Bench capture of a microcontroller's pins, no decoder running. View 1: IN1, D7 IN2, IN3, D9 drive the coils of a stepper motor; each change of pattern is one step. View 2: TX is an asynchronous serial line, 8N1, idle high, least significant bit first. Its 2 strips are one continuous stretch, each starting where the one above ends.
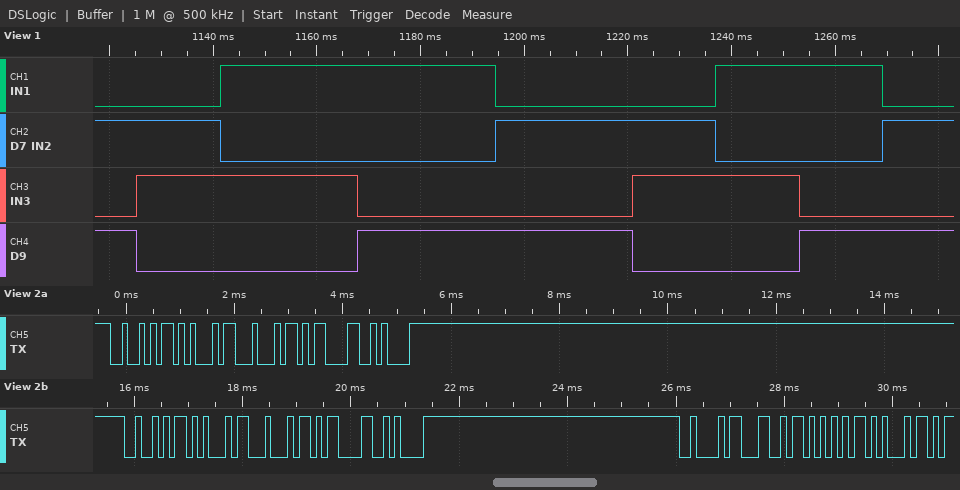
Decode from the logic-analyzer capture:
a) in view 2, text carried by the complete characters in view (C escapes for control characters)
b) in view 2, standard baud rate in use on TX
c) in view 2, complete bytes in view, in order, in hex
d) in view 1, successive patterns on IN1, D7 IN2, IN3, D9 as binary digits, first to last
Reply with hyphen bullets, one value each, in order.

- "RED\r\nRED\r\nBLUE"
- 9600 baud
- 52 45 44 0D 0A 52 45 44 0D 0A 42 4C 55 45
- 0101 0110 1010 1001 0101 0110 1010 1001 0101
